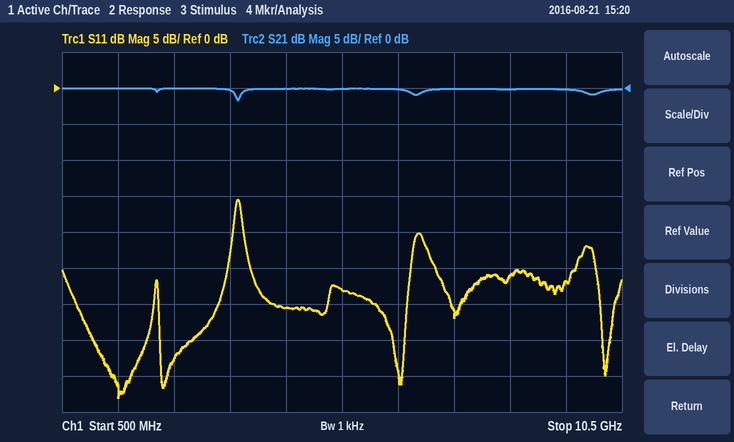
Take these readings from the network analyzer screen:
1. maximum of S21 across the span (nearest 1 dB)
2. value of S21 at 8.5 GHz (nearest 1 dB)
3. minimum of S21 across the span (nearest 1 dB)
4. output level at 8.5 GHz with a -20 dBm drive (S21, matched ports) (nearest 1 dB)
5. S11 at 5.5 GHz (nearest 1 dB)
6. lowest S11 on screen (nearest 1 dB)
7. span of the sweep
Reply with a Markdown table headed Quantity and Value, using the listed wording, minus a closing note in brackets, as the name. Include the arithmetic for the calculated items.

| Quantity | Value |
|---|---|
| maximum of S21 across the span | 0 dB |
| value of S21 at 8.5 GHz | 0 dB |
| minimum of S21 across the span | -2 dB |
| output level at 8.5 GHz with a -20 dBm drive (S21, matched ports) | -20 dBm + (0 dB) = -20 dBm |
| S11 at 5.5 GHz | -28 dB |
| lowest S11 on screen | -43 dB |
| span of the sweep | 10 GHz |
